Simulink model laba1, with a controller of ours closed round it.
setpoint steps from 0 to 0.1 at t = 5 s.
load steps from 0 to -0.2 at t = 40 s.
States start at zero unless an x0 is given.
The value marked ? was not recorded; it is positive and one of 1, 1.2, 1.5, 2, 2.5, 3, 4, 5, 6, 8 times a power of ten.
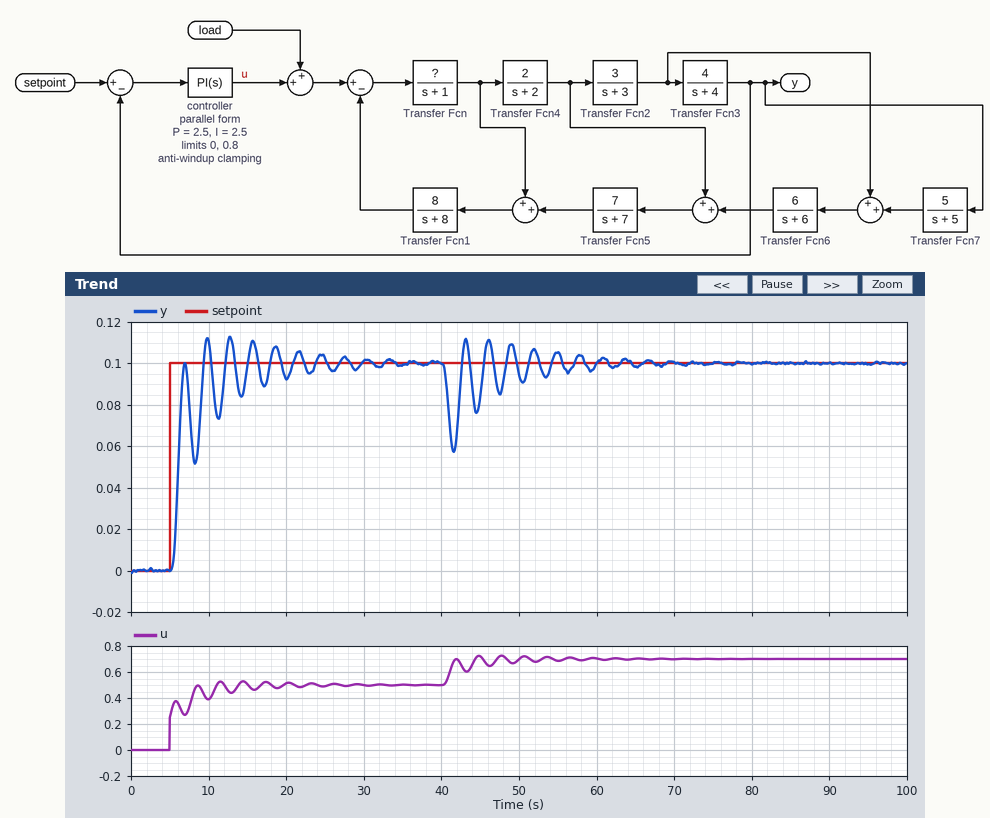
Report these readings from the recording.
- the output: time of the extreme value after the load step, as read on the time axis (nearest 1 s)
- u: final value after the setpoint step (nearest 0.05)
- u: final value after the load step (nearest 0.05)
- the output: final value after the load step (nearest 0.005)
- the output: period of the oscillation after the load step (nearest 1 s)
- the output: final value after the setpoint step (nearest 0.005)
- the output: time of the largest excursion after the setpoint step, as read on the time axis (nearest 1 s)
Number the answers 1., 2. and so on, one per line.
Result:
1. 42 s
2. 0.50
3. 0.70
4. 0.100
5. 3 s
6. 0.100
7. 13 s
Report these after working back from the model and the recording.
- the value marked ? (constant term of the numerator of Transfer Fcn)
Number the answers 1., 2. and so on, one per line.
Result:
1. 1
